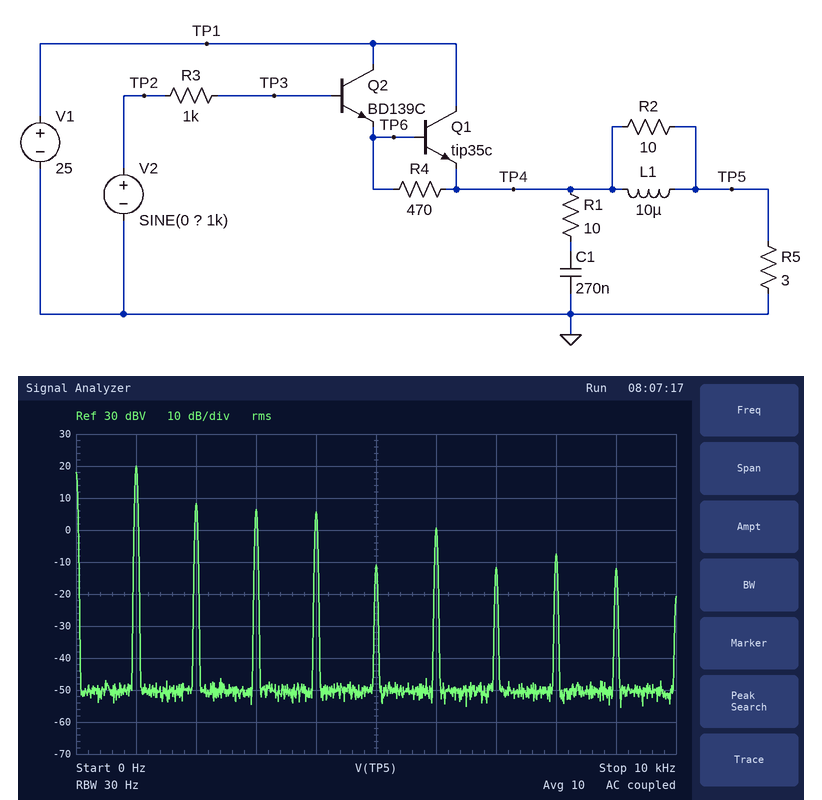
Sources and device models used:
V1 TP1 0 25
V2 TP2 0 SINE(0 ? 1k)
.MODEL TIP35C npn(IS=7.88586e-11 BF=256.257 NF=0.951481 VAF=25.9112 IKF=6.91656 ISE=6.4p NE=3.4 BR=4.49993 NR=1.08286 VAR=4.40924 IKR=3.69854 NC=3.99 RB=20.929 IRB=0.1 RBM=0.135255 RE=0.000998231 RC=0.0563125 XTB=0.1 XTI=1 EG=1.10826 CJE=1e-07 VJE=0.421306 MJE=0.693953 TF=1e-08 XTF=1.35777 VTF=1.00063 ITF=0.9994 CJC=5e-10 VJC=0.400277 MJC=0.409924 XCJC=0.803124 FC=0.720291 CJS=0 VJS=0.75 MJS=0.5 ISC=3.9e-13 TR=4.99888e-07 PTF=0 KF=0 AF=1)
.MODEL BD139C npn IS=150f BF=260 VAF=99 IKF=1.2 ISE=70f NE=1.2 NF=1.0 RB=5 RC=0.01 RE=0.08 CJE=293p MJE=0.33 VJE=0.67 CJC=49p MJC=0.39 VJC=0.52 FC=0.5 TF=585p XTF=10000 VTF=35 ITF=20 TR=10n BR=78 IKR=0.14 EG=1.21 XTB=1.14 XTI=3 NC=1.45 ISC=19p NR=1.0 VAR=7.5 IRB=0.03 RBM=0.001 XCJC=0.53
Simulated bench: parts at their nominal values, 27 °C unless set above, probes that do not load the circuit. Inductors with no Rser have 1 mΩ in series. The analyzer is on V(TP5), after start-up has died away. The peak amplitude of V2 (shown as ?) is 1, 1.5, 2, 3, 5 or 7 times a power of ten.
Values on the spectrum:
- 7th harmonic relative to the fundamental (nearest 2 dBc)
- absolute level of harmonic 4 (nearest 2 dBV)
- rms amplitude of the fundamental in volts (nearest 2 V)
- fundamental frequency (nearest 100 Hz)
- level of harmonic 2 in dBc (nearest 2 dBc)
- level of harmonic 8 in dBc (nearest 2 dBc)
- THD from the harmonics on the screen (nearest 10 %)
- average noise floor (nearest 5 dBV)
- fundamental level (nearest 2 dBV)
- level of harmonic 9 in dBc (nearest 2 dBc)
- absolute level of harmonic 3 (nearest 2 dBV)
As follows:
-32 dBc
6 dBV
10 V
1.0 kHz
-12 dBc
-28 dBc
40 %
-50 dBV
20 dBV
-32 dBc
6 dBV
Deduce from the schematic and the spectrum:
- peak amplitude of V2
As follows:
50 V
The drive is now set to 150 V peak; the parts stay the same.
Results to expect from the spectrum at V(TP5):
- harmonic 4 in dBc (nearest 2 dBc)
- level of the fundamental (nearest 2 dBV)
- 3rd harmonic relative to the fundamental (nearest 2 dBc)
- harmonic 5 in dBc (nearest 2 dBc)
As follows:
-22 dBc
20 dBV
-10 dBc
-16 dBc
